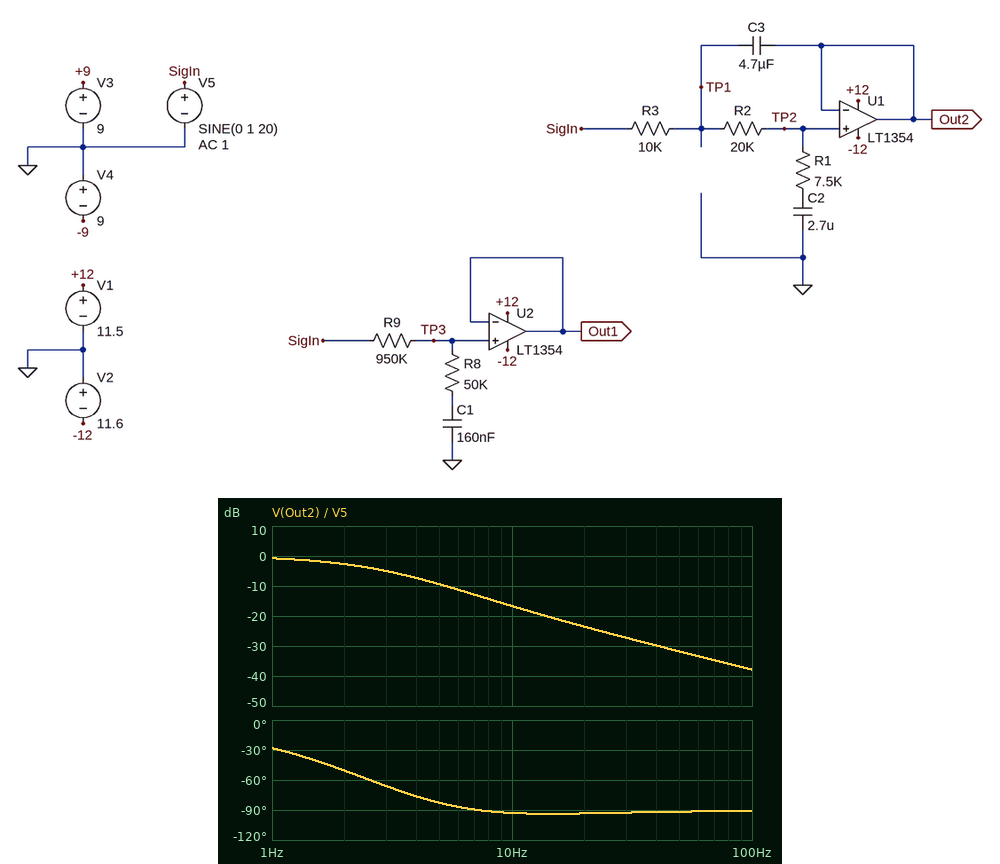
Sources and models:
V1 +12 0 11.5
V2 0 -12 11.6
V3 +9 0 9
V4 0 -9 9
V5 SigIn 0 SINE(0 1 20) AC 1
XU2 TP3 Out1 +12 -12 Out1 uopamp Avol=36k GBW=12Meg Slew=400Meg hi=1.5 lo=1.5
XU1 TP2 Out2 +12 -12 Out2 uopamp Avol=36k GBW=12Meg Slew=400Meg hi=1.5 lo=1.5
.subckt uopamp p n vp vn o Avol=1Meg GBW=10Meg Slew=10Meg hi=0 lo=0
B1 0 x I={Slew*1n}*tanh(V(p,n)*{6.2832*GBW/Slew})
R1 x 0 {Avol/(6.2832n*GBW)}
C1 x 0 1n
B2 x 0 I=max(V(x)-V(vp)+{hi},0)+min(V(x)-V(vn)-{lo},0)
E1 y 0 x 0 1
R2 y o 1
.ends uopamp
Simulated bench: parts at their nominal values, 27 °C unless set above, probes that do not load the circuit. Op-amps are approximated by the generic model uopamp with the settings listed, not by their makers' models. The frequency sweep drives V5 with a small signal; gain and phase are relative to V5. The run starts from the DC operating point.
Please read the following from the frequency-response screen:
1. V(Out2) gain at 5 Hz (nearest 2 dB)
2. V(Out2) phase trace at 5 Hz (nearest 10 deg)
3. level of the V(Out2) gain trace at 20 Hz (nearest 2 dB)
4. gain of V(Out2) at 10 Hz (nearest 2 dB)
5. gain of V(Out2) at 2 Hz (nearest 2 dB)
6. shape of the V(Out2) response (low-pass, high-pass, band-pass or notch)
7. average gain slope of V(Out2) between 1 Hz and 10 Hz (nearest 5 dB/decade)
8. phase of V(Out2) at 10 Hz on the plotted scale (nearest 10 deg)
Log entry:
-10 dB
-80 deg
-24 dB
-16 dB
-2 dB
low-pass
-15 dB/decade
-90 deg
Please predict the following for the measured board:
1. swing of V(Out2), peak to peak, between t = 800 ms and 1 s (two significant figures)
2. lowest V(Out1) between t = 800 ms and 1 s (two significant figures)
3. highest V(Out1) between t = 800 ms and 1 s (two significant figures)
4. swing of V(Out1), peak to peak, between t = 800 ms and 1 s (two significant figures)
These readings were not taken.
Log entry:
130 mV
-70 mV
71 mV
140 mV
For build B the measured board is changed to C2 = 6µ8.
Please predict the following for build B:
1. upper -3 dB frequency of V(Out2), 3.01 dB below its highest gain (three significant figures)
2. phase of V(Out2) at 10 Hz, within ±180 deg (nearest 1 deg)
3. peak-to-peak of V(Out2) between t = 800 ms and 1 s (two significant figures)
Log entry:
727 mHz
-74 deg
120 mV
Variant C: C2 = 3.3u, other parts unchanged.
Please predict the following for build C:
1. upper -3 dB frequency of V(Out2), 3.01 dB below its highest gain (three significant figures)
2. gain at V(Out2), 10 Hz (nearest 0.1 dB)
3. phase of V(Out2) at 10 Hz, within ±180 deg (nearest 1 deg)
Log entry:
1.68 Hz
-17.4 dB
-88 deg
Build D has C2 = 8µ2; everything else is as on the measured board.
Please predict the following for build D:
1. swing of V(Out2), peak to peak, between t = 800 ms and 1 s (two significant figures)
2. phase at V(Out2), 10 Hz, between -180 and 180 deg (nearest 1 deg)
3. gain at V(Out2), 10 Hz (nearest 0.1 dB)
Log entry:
120 mV
-71 deg
-18.9 dB
